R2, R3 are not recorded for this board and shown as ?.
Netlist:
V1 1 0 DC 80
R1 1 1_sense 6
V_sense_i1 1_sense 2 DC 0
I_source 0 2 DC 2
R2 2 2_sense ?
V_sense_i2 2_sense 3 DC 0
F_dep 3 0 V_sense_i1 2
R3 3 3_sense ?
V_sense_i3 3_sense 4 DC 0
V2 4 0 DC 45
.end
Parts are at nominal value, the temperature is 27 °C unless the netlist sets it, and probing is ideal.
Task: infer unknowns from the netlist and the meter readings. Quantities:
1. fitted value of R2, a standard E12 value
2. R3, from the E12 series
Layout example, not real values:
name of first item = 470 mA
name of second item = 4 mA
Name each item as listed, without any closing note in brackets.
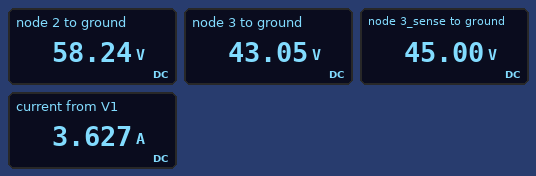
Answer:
fitted value of R2, a standard E12 value = 2.7 Ω
R3, from the E12 series = 1.2 Ω
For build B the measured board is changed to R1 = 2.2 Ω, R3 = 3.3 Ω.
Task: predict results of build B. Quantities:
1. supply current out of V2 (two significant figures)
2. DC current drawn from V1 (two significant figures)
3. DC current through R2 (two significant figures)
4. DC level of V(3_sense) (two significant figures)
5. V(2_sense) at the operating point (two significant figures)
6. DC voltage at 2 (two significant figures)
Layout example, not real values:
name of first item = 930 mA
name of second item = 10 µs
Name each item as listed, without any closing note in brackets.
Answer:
supply current out of V2 = 12 A
DC current drawn from V1 = 14 A
DC current through R2 = 16 A
DC level of V(3_sense) = 45 V
V(2_sense) at the operating point = 4.2 V
DC voltage at 2 = 48 V
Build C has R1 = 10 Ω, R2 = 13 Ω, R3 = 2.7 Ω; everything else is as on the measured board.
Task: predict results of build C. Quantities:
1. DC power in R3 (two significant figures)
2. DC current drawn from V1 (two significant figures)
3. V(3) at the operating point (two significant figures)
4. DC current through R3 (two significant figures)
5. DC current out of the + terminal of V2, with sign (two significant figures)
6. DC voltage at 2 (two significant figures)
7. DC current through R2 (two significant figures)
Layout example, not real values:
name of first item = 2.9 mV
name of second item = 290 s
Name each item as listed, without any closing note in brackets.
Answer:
DC power in R3 = 9.0 W
DC current drawn from V1 = 180 mA
V(3) at the operating point = 50 V
DC current through R3 = 1.8 A
DC current out of the + terminal of V2, with sign = -1.8 A
DC voltage at 2 = 78 V
DC current through R2 = 2.2 A
